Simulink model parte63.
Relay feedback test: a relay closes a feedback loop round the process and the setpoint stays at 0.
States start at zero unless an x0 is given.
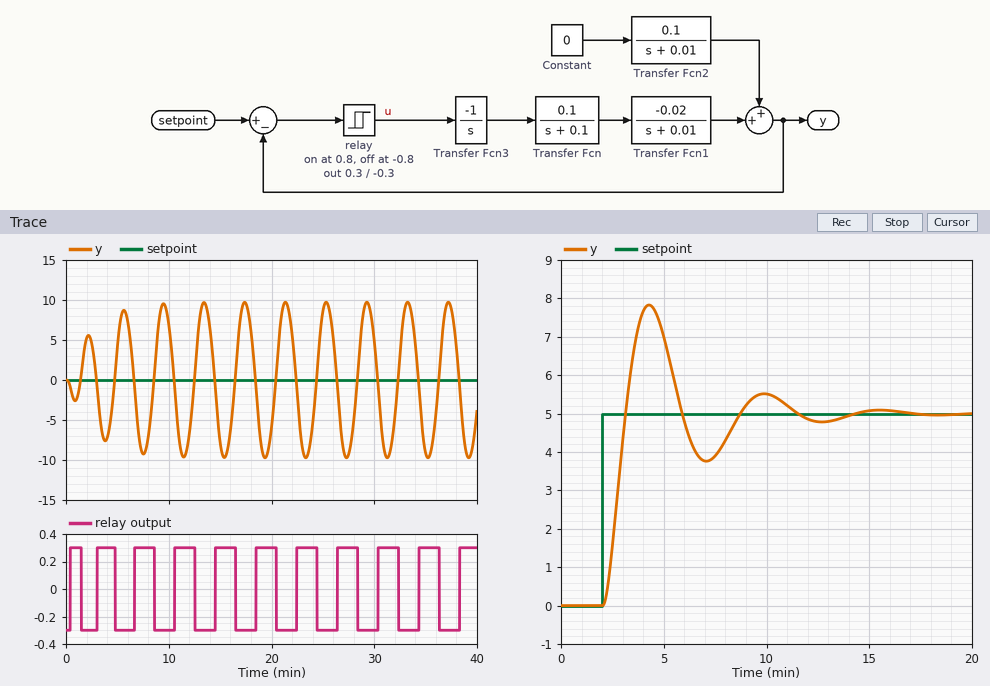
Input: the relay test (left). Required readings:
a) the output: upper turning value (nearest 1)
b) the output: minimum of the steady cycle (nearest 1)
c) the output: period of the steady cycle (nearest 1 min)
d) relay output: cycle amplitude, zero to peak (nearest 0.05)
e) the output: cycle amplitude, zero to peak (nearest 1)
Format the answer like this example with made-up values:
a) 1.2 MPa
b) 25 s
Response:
a) 10
b) -10
c) 4 min
d) 0.30
e) 10
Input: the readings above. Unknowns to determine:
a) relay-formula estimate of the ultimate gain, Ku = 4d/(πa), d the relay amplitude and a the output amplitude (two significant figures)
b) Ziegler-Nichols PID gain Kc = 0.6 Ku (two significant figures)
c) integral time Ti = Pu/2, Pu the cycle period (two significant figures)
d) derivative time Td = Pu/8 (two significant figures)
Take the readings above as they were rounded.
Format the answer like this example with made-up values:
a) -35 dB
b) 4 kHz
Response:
a) 0.038
b) 0.023
c) 2.0 min
d) 0.50 min
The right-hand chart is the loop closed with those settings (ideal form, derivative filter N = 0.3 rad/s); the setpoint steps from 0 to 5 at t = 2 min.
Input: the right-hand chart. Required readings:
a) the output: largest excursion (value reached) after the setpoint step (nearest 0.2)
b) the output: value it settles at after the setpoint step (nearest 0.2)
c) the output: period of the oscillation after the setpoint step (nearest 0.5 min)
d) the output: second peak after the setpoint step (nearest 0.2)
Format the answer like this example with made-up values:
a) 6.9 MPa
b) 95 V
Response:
a) 7.8
b) 5.0
c) 5.5 min
d) 5.6
